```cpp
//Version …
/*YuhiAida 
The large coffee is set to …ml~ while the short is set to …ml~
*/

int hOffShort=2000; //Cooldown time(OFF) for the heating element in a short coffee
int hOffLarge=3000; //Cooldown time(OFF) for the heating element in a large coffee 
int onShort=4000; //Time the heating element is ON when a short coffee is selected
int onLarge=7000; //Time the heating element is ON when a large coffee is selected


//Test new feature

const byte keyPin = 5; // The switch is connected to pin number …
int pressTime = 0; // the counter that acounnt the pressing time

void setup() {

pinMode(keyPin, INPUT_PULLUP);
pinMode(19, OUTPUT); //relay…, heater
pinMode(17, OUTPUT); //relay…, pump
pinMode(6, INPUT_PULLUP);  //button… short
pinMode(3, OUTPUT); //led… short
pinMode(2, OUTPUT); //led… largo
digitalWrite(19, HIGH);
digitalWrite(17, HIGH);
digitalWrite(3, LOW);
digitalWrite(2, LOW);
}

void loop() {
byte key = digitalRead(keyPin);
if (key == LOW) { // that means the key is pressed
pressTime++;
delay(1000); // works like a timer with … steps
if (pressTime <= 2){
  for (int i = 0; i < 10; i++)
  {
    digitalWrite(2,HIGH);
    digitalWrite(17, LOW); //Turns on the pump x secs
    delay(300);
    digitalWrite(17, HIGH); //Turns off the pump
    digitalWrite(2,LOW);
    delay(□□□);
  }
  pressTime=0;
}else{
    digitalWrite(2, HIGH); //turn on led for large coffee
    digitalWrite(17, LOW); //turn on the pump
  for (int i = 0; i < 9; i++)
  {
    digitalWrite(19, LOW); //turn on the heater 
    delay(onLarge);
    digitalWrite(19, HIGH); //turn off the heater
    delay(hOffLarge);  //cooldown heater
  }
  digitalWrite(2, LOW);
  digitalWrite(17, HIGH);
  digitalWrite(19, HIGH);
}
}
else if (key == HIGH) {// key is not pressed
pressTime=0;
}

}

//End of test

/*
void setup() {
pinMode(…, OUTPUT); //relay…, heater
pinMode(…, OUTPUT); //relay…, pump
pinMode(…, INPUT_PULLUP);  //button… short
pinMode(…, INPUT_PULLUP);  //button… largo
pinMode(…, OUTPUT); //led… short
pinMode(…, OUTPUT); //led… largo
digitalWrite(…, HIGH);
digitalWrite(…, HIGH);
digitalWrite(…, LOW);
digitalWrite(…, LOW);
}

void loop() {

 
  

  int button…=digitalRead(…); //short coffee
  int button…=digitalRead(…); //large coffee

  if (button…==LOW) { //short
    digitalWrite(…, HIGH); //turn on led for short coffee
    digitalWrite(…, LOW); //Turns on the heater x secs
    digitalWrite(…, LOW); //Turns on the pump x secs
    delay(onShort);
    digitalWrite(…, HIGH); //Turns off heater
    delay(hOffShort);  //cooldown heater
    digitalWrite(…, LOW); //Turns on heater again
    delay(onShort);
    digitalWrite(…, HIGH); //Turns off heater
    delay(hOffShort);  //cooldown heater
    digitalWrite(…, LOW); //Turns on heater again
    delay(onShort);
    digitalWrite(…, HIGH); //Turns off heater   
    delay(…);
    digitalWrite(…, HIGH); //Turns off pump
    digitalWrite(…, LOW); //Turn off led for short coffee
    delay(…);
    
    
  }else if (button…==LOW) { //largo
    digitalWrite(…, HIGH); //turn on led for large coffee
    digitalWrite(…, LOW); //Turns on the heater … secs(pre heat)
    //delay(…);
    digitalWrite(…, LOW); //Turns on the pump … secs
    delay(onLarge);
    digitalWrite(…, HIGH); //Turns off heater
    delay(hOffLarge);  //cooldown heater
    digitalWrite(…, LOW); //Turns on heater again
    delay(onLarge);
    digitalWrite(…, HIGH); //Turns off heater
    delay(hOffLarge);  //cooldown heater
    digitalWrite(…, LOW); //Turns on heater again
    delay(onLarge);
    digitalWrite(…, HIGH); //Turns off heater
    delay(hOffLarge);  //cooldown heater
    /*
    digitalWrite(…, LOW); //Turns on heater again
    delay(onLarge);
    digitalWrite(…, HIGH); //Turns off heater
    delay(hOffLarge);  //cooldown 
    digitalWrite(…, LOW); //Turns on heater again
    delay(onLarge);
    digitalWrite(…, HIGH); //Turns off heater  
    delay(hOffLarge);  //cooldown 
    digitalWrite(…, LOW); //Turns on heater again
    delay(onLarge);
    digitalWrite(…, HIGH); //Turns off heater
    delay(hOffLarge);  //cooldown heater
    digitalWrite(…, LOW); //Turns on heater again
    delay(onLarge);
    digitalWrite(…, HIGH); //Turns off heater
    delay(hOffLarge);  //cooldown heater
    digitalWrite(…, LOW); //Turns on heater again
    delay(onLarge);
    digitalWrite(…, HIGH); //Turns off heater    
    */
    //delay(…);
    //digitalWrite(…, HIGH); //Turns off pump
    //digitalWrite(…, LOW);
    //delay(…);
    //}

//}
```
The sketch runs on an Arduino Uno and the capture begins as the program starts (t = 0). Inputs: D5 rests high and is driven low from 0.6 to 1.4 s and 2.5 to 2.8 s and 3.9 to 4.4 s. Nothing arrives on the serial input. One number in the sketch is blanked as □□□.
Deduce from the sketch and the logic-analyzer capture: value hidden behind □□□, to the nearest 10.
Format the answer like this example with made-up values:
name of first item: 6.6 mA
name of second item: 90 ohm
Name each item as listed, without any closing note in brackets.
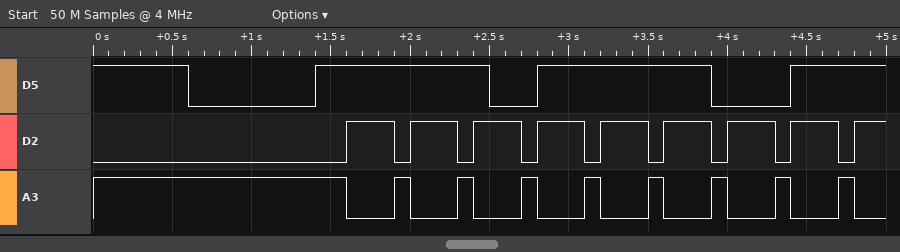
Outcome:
value hidden behind □□□, to the nearest 10: 100
